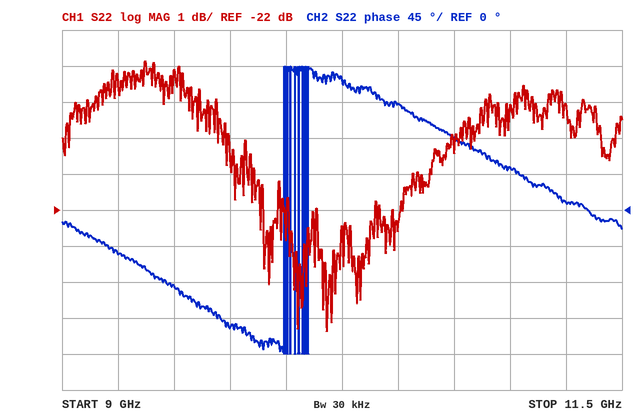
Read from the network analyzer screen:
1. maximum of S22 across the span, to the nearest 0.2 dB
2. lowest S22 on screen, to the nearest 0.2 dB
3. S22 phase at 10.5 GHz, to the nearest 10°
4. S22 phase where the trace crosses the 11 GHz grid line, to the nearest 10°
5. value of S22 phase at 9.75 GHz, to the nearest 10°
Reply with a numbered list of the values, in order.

1. -17.8 dB
2. -25.4 dB
3. 130°
4. 50°
5. -150°
